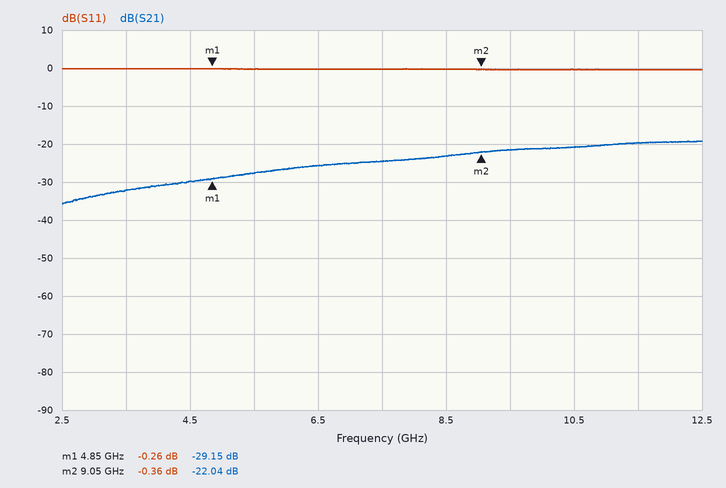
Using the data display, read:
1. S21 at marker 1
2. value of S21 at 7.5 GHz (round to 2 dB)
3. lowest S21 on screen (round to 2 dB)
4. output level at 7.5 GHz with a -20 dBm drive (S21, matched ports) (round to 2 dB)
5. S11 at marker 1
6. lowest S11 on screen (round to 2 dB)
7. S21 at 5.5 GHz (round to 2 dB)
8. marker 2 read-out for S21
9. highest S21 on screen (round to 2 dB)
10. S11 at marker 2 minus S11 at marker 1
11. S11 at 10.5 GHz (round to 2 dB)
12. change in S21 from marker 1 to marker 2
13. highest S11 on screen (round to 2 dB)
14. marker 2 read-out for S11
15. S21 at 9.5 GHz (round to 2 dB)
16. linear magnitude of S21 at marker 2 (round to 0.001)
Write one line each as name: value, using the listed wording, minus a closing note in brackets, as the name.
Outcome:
S21 at marker 1: -29.15 dB
value of S21 at 7.5 GHz: -24 dB
lowest S21 on screen: -36 dB
output level at 7.5 GHz with a -20 dBm drive (S21, matched ports): -44 dBm
S11 at marker 1: -0.26 dB
lowest S11 on screen: 0 dB
S21 at 5.5 GHz: -28 dB
marker 2 read-out for S21: -22.04 dB
highest S21 on screen: -20 dB
S11 at marker 2 minus S11 at marker 1: -0.10 dB
S11 at 10.5 GHz: 0 dB
change in S21 from marker 1 to marker 2: 7.11 dB
highest S11 on screen: 0 dB
marker 2 read-out for S11: -0.36 dB
S21 at 9.5 GHz: -22 dB
linear magnitude of S21 at marker 2: 0.079
